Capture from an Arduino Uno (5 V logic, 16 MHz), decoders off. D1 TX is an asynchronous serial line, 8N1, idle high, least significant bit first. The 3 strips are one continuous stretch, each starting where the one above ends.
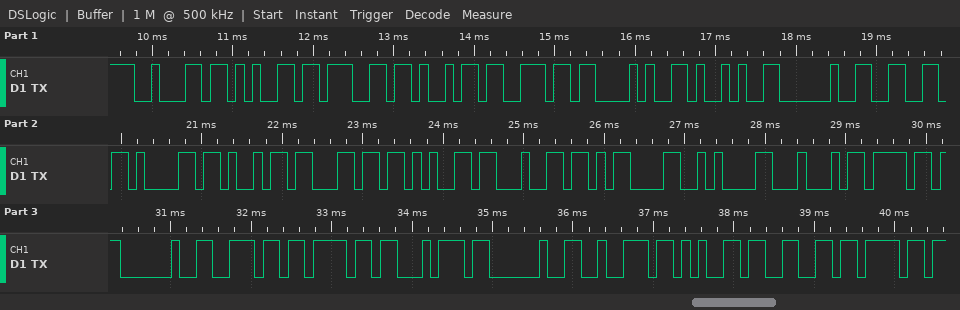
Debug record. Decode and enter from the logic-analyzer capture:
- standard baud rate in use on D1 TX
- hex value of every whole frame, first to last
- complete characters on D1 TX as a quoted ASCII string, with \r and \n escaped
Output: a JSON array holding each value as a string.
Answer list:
["9600 baud", "0x62 0x65 0x67 0x69 0x6E 0x28 0x29 0x20 0x66 0x61 0x69 0x6C 0x65 0x64 0x0D 0x0A 0x44 0x6F 0x20 0x6E 0x6F 0x74 0x20 0x72 0x65 0x66 0x6F", "\"begin() failed\\r\\nDo not refo\""]
